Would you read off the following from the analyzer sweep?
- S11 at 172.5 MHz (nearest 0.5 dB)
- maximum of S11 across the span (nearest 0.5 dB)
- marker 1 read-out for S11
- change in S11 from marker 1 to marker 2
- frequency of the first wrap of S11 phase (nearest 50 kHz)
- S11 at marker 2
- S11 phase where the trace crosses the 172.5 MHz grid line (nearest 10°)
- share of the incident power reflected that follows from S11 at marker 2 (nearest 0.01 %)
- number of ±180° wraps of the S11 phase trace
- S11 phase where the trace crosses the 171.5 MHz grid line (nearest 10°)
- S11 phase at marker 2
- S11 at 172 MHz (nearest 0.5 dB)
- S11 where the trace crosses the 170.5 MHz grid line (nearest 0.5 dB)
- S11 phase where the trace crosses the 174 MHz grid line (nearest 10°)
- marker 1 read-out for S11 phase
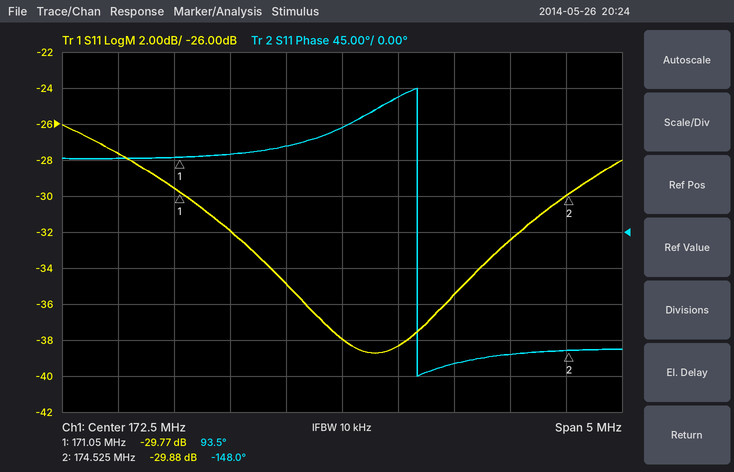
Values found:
-38.0 dB
-26.0 dB
-29.77 dB
-0.11 dB
173.15 MHz
-29.88 dB
130°
0.10 %
1
100°
-148.0°
-35.0 dB
-27.5 dB
-150°
93.5°
